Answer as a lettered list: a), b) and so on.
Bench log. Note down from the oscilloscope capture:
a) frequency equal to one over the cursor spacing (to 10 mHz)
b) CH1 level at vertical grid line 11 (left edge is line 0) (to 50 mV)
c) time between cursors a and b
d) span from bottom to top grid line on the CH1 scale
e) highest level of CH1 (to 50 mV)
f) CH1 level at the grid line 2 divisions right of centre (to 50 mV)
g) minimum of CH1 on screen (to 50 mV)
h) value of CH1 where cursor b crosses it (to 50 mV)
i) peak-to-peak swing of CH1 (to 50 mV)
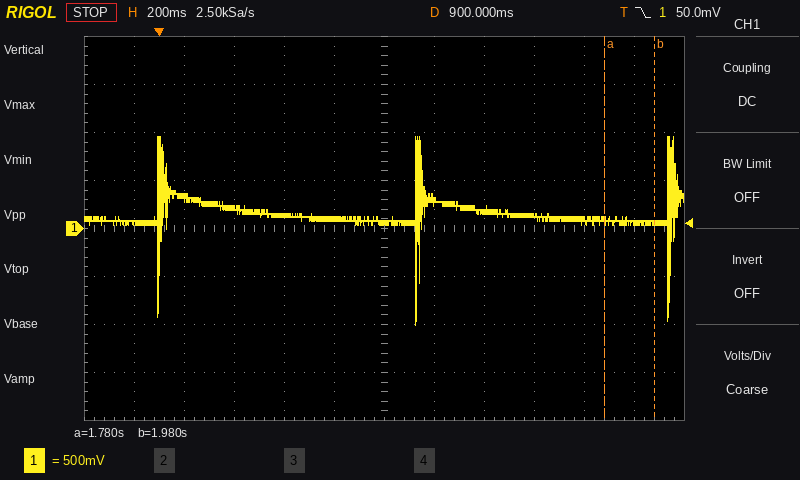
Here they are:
a) 5.00 Hz
b) 50 mV
c) 200 ms
d) 4 V
e) 950 mV
f) 200 mV
g) -1.00 V
h) 50 mV
i) 1.95 V
